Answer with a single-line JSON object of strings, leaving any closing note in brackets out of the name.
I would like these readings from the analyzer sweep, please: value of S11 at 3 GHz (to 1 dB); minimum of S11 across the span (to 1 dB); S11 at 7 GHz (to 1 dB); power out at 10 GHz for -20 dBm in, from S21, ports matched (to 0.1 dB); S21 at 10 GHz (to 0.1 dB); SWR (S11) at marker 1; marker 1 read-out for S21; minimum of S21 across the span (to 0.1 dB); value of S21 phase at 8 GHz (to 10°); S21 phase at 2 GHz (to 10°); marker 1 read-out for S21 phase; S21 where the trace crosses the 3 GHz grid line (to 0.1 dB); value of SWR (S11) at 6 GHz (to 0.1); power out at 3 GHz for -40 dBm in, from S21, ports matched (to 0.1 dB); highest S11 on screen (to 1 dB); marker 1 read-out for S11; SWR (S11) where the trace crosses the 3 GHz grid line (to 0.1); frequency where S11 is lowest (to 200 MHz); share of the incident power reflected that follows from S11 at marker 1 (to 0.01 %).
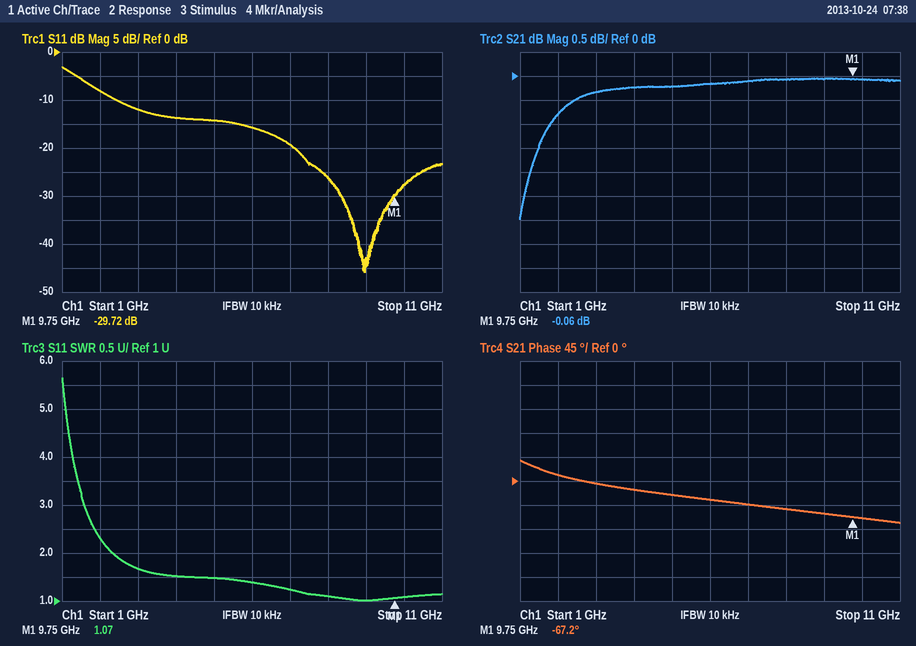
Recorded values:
{"value of S11 at 3 GHz": "-12 dB", "minimum of S11 across the span": "-46 dB", "S11 at 7 GHz": "-19 dB", "power out at 10 GHz for -20 dBm in, from S21, ports matched": "-20.1 dBm", "S21 at 10 GHz": "-0.1 dB", "SWR (S11) at marker 1": "1.07", "marker 1 read-out for S21": "-0.06 dB", "minimum of S21 across the span": "-3.0 dB", "value of S21 phase at 8 GHz": "-50°", "S21 phase at 2 GHz": "10°", "marker 1 read-out for S21 phase": "-67.2°", "S21 where the trace crosses the 3 GHz grid line": "-0.3 dB", "value of SWR (S11) at 6 GHz": "1.4", "power out at 3 GHz for -40 dBm in, from S21, ports matched": "-40.3 dBm", "highest S11 on screen": "-3 dB", "marker 1 read-out for S11": "-29.72 dB", "SWR (S11) where the trace crosses the 3 GHz grid line": "1.7", "frequency where S11 is lowest": "9.0 GHz", "share of the incident power reflected that follows from S11 at marker 1": "0.11 %"}
